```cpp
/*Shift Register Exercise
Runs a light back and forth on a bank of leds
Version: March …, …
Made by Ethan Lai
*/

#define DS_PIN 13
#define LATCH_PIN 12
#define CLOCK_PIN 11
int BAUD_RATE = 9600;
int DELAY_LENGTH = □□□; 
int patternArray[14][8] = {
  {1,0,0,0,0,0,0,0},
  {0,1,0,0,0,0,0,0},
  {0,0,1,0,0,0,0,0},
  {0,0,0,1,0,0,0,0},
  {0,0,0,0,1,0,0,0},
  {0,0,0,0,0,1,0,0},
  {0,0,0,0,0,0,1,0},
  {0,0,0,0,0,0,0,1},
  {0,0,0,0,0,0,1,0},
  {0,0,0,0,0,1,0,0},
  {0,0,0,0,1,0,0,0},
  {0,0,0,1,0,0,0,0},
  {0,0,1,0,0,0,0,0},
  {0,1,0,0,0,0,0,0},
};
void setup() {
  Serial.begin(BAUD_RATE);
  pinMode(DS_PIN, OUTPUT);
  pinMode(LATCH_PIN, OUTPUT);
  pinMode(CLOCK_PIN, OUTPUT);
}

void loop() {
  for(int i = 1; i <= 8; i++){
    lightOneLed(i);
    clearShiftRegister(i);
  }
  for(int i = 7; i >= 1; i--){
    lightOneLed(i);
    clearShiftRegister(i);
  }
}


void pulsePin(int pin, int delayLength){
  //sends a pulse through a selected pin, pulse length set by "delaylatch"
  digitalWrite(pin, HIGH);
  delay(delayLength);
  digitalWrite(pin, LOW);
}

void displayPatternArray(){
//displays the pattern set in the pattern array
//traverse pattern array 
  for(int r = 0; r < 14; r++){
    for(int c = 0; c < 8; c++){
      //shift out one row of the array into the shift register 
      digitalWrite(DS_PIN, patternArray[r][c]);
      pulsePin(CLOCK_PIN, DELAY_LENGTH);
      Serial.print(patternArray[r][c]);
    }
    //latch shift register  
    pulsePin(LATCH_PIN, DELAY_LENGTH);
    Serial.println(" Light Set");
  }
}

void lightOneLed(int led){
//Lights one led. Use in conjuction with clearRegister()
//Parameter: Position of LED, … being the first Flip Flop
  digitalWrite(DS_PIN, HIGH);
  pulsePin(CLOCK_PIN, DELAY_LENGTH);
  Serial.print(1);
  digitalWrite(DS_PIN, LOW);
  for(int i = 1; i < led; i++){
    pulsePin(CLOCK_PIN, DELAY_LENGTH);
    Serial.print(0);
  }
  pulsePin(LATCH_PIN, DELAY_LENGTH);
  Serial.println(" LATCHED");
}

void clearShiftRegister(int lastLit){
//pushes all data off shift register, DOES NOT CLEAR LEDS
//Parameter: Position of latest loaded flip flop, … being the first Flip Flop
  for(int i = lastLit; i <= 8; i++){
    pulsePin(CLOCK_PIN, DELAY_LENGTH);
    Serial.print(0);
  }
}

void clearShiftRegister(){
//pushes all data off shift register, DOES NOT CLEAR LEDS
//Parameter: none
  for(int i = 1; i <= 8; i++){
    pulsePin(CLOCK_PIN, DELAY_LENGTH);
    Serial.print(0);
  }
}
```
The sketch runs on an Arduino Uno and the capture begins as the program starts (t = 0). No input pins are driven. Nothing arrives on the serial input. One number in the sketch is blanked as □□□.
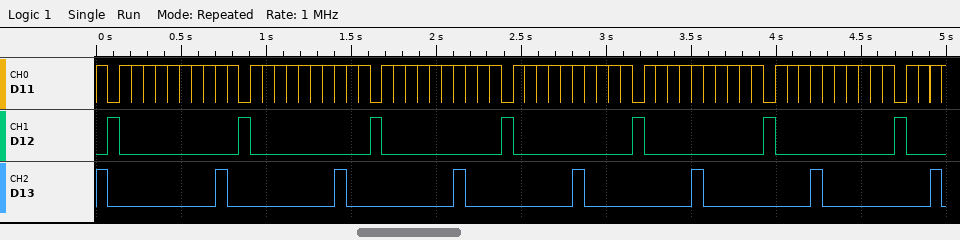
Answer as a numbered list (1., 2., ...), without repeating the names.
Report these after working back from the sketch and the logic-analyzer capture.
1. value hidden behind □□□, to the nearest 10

1. 70
